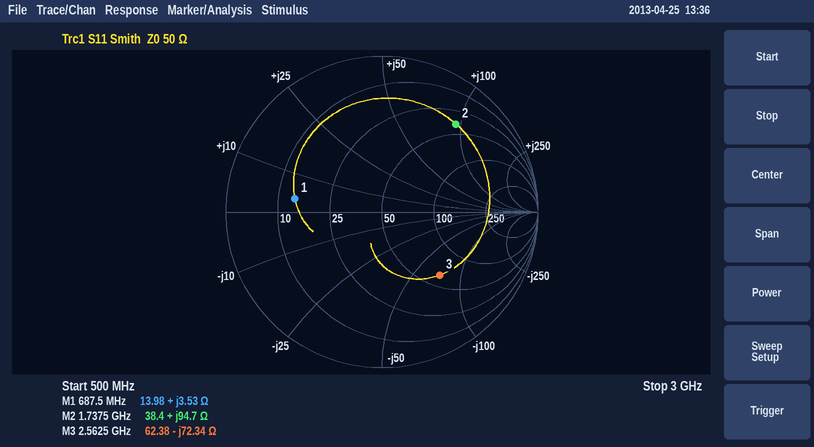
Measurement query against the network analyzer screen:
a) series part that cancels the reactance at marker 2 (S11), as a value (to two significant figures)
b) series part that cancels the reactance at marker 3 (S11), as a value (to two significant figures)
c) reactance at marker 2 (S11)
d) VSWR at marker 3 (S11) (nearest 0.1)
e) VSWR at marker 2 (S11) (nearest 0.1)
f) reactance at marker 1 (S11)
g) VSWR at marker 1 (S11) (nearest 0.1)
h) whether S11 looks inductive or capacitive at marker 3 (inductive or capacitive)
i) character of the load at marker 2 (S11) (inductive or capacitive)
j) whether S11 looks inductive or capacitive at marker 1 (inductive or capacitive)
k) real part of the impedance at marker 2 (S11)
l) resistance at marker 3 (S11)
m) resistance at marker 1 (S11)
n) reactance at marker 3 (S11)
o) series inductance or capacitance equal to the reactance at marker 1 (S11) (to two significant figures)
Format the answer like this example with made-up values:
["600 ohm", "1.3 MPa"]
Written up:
["970 fF", "4.5 nH", "+94.7 Ω", "3.4", "6.6", "+3.53 Ω", "3.6", "capacitive", "inductive", "inductive", "38.4 Ω", "62.38 Ω", "13.98 Ω", "-72.34 Ω", "820 pH"]
